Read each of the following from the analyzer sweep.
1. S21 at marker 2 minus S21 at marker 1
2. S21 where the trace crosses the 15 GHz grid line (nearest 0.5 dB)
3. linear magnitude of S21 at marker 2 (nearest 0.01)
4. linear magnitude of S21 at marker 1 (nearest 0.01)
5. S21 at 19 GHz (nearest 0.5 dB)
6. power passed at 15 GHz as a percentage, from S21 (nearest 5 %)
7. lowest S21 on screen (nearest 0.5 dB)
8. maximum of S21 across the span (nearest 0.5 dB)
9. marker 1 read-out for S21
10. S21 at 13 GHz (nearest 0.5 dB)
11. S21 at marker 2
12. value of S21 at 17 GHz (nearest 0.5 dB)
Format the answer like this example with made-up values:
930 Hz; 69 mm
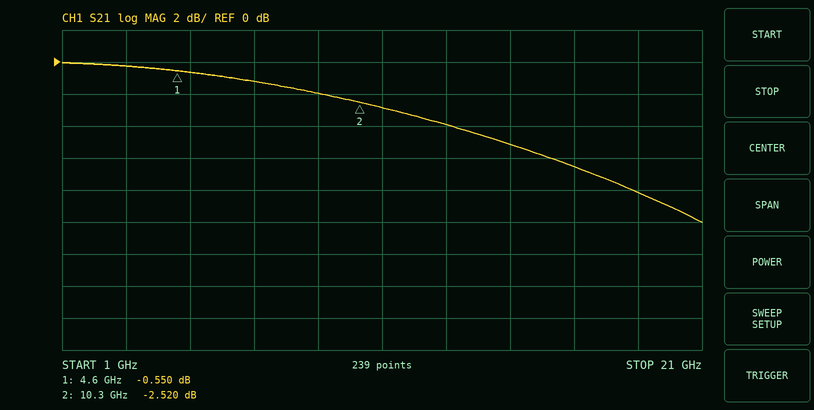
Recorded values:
-1.970 dB; -5.0 dB; 0.75; 0.94; -8.0 dB; 30 %; -10.0 dB; 0.0 dB; -0.550 dB; -4.0 dB; -2.520 dB; -6.5 dB
